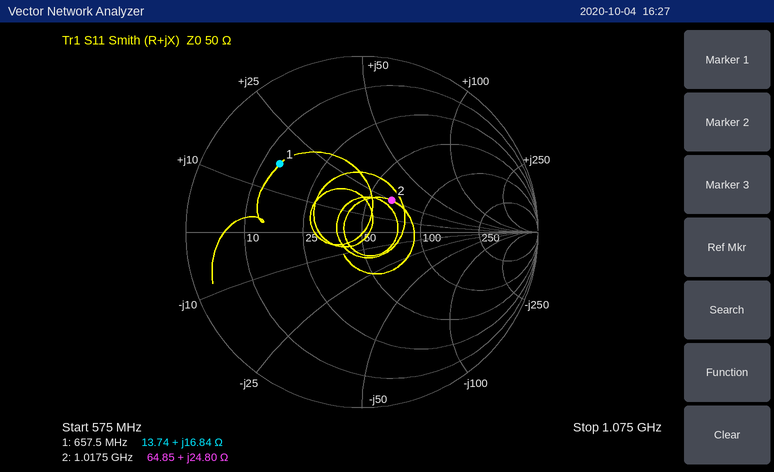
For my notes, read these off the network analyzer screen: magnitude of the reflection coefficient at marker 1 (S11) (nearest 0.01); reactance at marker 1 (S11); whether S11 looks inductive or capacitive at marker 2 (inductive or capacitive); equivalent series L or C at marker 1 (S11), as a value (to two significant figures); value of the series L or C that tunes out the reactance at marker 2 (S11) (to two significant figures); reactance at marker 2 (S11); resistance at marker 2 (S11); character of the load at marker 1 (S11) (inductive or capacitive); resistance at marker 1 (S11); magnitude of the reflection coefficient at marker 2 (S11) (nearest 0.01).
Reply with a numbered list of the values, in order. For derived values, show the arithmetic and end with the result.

1. 0.61
2. +16.84 Ω
3. inductive
4. L = 16.84 Ω/(2π × 657.5 MHz) ≈ 4.1 nH
5. C = 1/(2π × 1.0175 GHz × 24.8 Ω) ≈ 6.3 pF
6. +24.80 Ω
7. 64.85 Ω
8. inductive
9. 13.74 Ω
10. 0.25
